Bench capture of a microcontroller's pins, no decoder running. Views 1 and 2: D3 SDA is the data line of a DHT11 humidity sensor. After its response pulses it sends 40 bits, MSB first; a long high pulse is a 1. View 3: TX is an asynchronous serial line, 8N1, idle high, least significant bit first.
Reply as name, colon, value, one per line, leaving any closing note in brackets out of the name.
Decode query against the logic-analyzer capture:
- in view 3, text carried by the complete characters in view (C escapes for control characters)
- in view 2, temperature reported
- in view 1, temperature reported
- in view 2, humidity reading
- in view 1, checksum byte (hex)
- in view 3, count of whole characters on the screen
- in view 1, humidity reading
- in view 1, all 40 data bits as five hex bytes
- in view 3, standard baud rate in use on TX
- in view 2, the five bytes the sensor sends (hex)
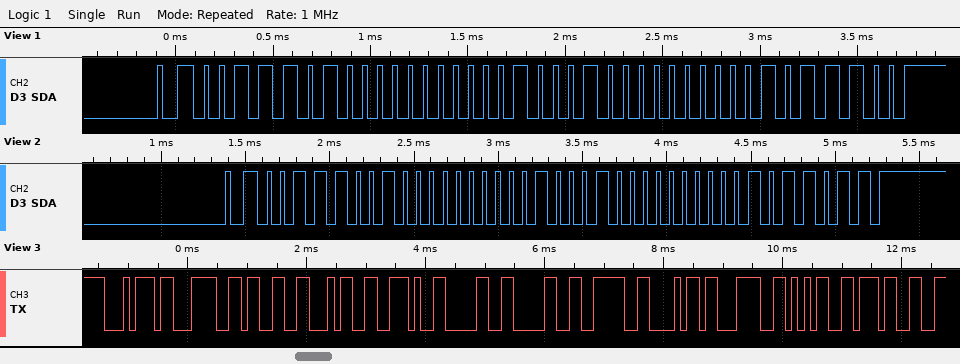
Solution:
in view 3, text carried by the complete characters in view: "t<34.00>h<57"
in view 2, temperature reported: 34.0 °C
in view 1, temperature reported: 34.0 °C
in view 2, humidity reading: 57 %
in view 1, checksum byte: 0x5C
in view 3, count of whole characters on the screen: 12
in view 1, humidity reading: 58 %
in view 1, all 40 data bits as five hex bytes: 3A 00 22 00 5C
in view 3, standard baud rate in use on TX: 9600 baud
in view 2, the five bytes the sensor sends: 39 00 22 00 5B
